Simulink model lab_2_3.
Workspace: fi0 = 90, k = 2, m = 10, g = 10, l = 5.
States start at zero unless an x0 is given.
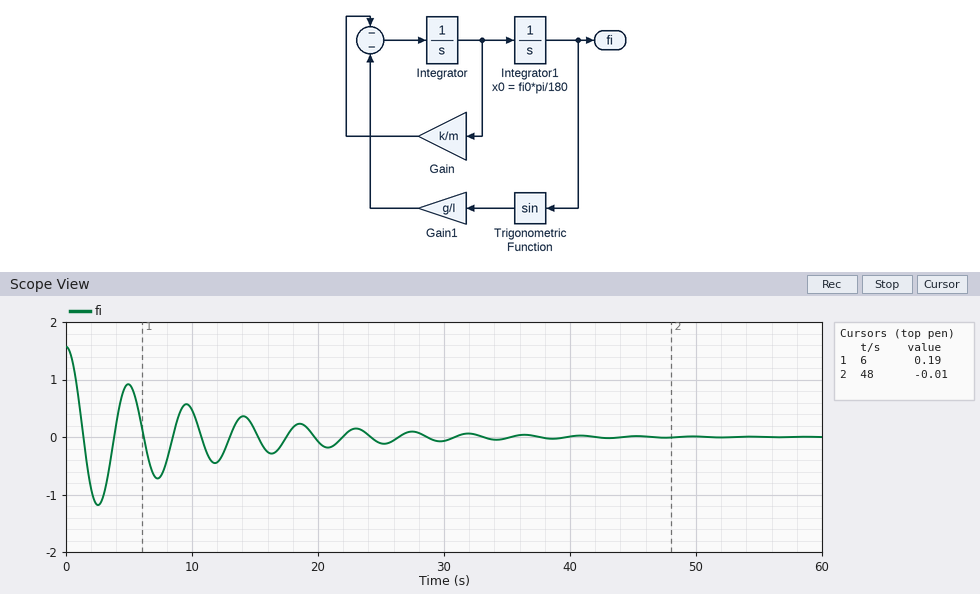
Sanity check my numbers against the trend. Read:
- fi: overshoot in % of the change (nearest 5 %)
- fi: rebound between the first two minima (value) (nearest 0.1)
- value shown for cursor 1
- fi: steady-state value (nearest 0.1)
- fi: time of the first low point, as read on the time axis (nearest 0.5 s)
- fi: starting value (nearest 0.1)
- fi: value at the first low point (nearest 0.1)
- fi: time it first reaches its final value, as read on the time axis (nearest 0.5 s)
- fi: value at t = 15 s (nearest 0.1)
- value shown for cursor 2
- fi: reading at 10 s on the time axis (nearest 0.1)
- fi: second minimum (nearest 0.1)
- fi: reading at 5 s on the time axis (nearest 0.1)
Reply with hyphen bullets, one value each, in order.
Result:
- 75 %
- 0.9
- 0.19
- 0.0
- 2.5 s
- 1.6
- -1.2
- 1.5 s
- 0.1
- -0.01
- 0.5
- -0.7
- 0.9
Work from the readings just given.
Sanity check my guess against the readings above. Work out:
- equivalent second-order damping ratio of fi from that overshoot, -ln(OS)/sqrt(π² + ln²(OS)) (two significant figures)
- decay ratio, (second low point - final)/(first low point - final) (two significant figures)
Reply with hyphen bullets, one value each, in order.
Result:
- 0.091
- 0.58
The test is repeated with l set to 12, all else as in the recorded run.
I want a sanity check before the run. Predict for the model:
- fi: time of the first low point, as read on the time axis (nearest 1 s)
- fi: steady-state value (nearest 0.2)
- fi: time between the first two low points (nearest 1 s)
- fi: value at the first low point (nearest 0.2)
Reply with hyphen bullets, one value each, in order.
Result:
- 4 s
- 0.0
- 7 s
- -1.0
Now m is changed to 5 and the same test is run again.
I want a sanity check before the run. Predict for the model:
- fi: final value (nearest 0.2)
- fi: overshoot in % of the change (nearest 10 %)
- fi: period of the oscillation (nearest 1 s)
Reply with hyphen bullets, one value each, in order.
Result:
- 0.0
- 60 %
- 5 s
